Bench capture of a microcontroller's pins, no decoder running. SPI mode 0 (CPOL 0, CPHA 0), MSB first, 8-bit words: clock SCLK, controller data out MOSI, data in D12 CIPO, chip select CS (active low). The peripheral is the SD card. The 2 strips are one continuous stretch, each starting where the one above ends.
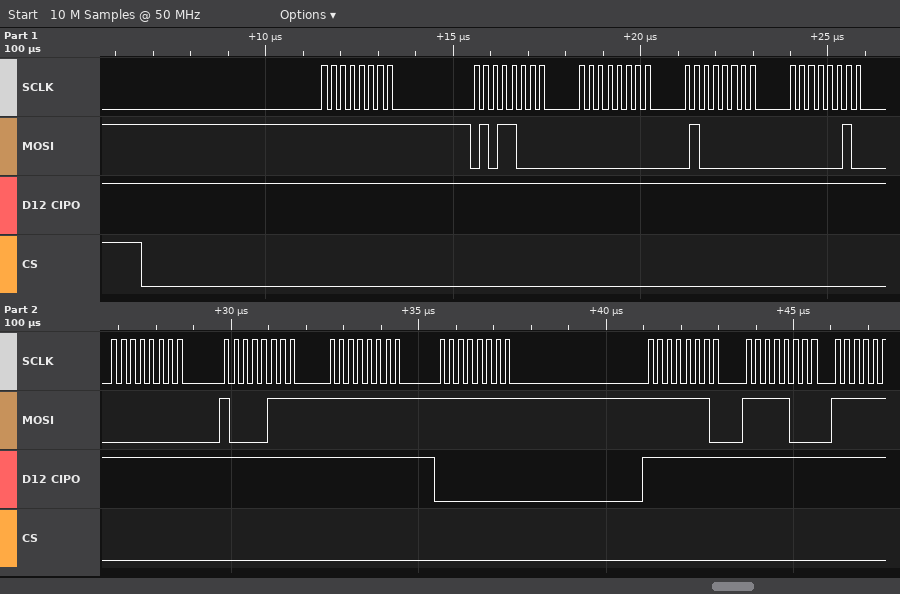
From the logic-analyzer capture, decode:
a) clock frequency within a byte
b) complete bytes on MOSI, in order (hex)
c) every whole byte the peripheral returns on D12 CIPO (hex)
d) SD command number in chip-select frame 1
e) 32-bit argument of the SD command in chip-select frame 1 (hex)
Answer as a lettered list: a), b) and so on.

a) 4 MHz
b) FF 58 00 40 02 00 87 FF FF FE F8
c) FF FF FF FF FF FF FF FF 00 FF FF
d) CMD24
e) 0x00400200
